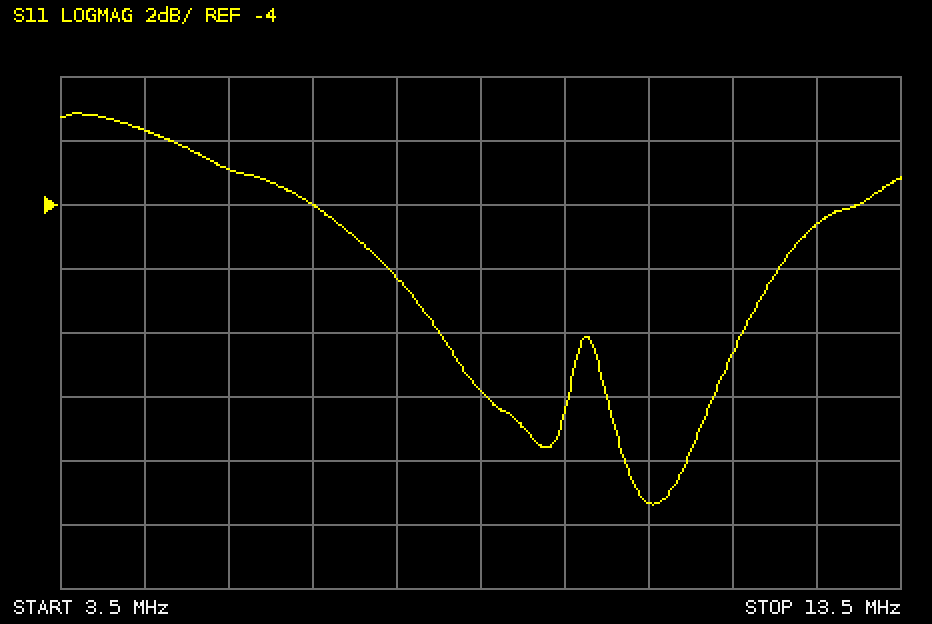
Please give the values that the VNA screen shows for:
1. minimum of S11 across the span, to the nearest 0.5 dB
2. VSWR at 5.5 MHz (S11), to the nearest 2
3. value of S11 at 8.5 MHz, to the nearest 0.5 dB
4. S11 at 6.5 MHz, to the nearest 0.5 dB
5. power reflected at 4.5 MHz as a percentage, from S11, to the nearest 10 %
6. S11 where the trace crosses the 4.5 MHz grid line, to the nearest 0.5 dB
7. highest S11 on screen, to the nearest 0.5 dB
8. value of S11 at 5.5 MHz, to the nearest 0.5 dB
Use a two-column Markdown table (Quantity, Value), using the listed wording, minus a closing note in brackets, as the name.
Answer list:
| Quantity | Value |
|---|---|
| minimum of S11 across the span, to the nearest 0.5 dB | -13.5 dB |
| VSWR at 5.5 MHz (S11), to the nearest 2 | 6 |
| value of S11 at 8.5 MHz, to the nearest 0.5 dB | -10.0 dB |
| S11 at 6.5 MHz, to the nearest 0.5 dB | -4.0 dB |
| power reflected at 4.5 MHz as a percentage, from S11, to the nearest 10 % | 70 % |
| S11 where the trace crosses the 4.5 MHz grid line, to the nearest 0.5 dB | -1.5 dB |
| highest S11 on screen, to the nearest 0.5 dB | -1.0 dB |
| value of S11 at 5.5 MHz, to the nearest 0.5 dB | -3.0 dB |
